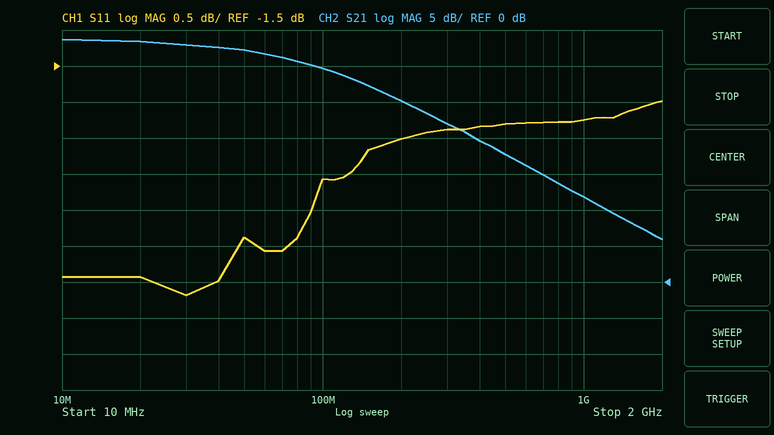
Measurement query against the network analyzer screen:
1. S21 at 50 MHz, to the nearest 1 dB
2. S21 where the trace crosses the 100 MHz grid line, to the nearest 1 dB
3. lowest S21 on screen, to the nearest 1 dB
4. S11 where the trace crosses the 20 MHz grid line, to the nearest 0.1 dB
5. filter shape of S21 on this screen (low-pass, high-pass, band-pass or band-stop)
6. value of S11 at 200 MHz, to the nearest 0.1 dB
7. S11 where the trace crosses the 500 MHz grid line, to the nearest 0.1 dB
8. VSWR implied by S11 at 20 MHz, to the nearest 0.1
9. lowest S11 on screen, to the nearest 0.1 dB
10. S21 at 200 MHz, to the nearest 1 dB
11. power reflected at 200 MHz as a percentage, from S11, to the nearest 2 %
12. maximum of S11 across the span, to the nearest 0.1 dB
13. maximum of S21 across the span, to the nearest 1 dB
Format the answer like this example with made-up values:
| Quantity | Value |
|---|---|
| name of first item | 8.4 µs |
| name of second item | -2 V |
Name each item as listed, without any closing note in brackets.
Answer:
| Quantity | Value |
|---|---|
| S21 at 50 MHz, to the nearest 1 dB | 32 dB |
| S21 where the trace crosses the 100 MHz grid line, to the nearest 1 dB | 30 dB |
| lowest S21 on screen, to the nearest 1 dB | 6 dB |
| S11 where the trace crosses the 20 MHz grid line, to the nearest 0.1 dB | -4.4 dB |
| filter shape of S21 on this screen | low-pass |
| value of S11 at 200 MHz, to the nearest 0.1 dB | -2.5 dB |
| S11 where the trace crosses the 500 MHz grid line, to the nearest 0.1 dB | -2.3 dB |
| VSWR implied by S11 at 20 MHz, to the nearest 0.1 | 4.0 |
| lowest S11 on screen, to the nearest 0.1 dB | -4.7 dB |
| S21 at 200 MHz, to the nearest 1 dB | 25 dB |
| power reflected at 200 MHz as a percentage, from S11, to the nearest 2 % | 56 % |
| maximum of S11 across the span, to the nearest 0.1 dB | -2.0 dB |
| maximum of S21 across the span, to the nearest 1 dB | 34 dB |
